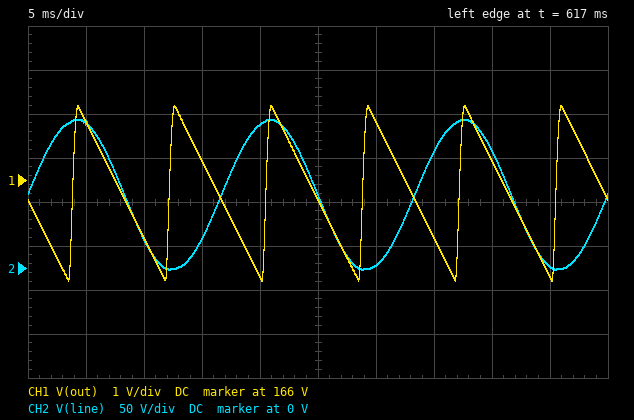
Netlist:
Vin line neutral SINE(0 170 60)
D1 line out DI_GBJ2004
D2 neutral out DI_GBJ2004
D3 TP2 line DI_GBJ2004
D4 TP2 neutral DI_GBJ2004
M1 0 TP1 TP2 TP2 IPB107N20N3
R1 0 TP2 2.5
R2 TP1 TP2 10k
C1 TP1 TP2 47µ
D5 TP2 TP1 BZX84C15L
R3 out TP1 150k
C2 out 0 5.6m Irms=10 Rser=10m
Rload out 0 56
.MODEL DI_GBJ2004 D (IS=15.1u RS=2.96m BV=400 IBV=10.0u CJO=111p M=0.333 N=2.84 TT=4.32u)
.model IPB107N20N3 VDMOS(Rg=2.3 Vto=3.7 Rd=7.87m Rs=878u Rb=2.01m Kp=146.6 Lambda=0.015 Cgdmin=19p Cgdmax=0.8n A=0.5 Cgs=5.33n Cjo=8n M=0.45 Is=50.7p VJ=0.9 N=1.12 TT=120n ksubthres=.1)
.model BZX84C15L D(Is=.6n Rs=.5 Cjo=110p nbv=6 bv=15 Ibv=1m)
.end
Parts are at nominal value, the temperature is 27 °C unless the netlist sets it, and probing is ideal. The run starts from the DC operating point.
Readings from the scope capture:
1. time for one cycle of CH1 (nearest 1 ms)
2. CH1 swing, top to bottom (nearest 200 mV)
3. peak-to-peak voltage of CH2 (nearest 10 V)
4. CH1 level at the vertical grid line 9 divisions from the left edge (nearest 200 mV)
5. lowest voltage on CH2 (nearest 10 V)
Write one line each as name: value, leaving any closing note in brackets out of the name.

time for one cycle of CH1: 8 ms
CH1 swing, top to bottom: 4.0 V
peak-to-peak voltage of CH2: 170 V
CH1 level at the vertical grid line 9 divisions from the left edge: 163.8 V
lowest voltage on CH2: 0 V
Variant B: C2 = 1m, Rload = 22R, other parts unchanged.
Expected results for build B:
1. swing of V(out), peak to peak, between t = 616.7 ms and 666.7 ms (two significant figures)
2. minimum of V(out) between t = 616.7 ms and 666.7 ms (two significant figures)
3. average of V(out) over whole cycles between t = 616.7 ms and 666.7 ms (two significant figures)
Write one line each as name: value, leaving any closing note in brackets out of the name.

swing of V(out), peak to peak, between t = 616.7 ms and 666.7 ms: 41 V
minimum of V(out) between t = 616.7 ms and 666.7 ms: 130 V
average of V(out) over whole cycles between t = 616.7 ms and 666.7 ms: 150 V
